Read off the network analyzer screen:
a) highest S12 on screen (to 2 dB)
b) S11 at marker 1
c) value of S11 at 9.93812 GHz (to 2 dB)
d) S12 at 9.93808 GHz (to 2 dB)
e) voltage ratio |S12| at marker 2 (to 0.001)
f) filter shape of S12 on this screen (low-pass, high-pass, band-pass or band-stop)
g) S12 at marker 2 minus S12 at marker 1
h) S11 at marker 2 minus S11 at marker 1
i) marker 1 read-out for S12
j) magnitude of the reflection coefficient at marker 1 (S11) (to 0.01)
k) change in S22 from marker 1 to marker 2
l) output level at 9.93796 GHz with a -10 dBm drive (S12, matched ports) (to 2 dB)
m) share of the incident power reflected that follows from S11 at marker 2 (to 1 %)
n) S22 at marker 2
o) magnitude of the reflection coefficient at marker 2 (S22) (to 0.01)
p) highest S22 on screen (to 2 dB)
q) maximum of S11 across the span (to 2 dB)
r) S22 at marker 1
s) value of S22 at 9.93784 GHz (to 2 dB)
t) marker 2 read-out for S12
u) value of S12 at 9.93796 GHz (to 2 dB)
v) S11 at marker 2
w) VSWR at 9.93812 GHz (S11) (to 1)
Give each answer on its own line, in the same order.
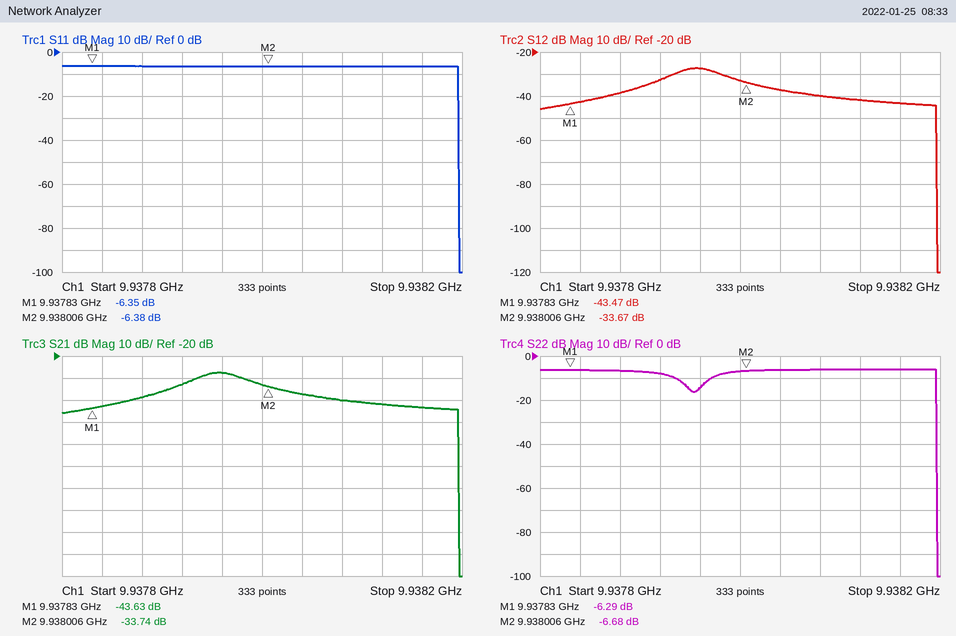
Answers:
-28 dB
-6.35 dB
-6 dB
-40 dB
0.021
band-pass
9.80 dB
-0.03 dB
-43.47 dB
0.48
-0.39 dB
-38 dBm
23 %
-6.68 dB
0.46
-6 dB
-6 dB
-6.29 dB
-6 dB
-33.67 dB
-28 dB
-6.38 dB
3
